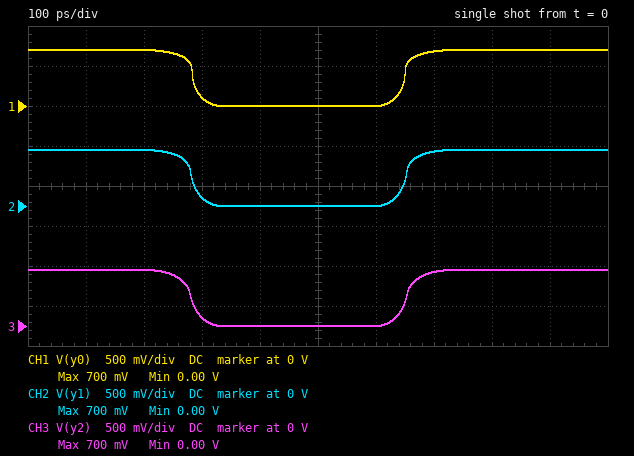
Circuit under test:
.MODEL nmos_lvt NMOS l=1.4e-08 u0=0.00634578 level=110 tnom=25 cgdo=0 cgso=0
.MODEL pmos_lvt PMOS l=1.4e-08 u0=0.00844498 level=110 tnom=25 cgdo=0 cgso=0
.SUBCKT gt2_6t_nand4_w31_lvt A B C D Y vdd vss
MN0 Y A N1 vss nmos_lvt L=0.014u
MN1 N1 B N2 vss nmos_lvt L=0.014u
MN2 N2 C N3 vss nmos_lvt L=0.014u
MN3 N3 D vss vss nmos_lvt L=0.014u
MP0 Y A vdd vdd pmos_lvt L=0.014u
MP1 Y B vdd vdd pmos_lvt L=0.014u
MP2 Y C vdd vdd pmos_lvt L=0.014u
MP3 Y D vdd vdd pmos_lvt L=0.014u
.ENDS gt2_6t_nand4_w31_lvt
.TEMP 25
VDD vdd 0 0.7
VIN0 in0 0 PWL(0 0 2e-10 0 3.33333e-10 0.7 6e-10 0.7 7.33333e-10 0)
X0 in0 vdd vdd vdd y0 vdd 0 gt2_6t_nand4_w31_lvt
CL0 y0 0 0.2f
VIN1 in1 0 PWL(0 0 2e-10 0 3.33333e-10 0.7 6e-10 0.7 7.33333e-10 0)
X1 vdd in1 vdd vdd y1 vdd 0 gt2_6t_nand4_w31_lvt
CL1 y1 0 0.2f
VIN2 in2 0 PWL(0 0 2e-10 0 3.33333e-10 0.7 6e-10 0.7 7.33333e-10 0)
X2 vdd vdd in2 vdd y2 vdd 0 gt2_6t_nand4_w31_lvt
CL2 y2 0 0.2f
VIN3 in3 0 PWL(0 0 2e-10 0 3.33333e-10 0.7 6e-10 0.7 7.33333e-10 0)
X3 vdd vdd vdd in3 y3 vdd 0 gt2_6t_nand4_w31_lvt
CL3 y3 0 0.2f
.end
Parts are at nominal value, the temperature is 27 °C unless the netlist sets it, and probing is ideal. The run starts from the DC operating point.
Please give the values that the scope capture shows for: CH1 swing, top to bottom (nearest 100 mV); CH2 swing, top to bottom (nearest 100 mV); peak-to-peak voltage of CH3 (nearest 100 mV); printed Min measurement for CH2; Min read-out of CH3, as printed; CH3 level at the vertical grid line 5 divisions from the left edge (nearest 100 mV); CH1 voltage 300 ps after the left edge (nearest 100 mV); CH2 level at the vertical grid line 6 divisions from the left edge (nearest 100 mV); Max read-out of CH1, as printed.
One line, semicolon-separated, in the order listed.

700 mV; 700 mV; 700 mV; 0.00 V; 0.00 V; 0 V; 100 mV; 0 V; 700 mV
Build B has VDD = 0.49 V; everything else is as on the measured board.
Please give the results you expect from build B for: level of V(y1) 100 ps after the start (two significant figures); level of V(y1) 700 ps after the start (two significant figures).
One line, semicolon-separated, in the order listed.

490 mV; 460 mV
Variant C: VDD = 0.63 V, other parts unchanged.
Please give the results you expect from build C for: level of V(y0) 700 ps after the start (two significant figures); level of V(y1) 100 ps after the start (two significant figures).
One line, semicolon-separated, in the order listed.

610 mV; 630 mV
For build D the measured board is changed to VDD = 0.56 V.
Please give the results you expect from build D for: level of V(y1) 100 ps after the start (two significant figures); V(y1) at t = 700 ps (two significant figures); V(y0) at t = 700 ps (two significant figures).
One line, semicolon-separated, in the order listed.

560 mV; 530 mV; 540 mV
